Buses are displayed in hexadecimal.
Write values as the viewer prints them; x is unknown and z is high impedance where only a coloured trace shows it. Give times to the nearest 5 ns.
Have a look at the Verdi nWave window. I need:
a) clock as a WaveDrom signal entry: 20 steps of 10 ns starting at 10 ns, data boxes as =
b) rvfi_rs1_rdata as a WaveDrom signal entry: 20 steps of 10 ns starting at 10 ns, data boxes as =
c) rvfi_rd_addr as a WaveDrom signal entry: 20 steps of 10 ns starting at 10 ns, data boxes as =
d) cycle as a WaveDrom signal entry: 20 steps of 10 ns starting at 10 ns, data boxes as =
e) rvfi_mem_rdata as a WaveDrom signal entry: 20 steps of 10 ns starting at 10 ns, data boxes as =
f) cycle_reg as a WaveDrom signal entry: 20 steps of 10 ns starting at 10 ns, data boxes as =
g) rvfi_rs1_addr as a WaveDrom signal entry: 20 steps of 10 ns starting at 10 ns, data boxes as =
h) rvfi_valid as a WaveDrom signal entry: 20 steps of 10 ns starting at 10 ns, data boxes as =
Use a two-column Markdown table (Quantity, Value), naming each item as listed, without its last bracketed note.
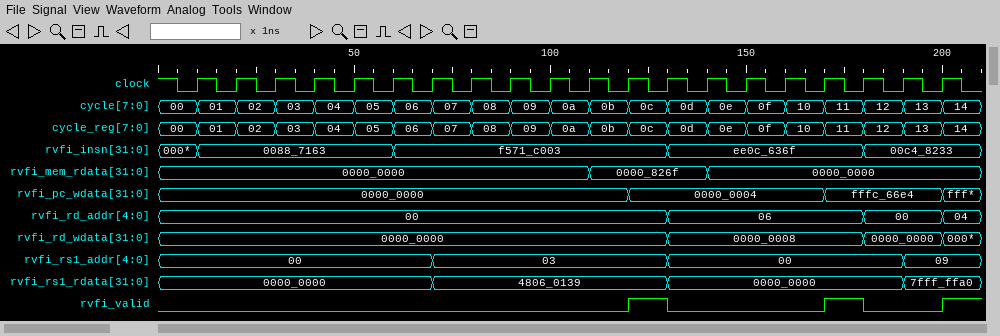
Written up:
| Quantity | Value |
|---|---|
| clock as a WaveDrom signal entry: 20 steps of 10 ns starting at 10 ns, data boxes as = | {name: 'clock', wave: 'p...................'} |
| rvfi_rs1_rdata as a WaveDrom signal entry: 20 steps of 10 ns starting at 10 ns, data boxes as = | {name: 'rvfi_rs1_rdata', wave: '=.....=.....=.....=.', data: '0000_0000 4806_0139 0000_0000 7fff_ffa0'} |
| rvfi_rd_addr as a WaveDrom signal entry: 20 steps of 10 ns starting at 10 ns, data boxes as = | {name: 'rvfi_rd_addr', wave: '=...........=....=.=', data: '00 06 00 04'} |
| cycle as a WaveDrom signal entry: 20 steps of 10 ns starting at 10 ns, data boxes as = | {name: 'cycle', wave: '====================', data: '01 02 03 04 05 06 07 08 09 0a 0b 0c 0d 0e 0f 10 11 12 13 14'} |
| rvfi_mem_rdata as a WaveDrom signal entry: 20 steps of 10 ns starting at 10 ns, data boxes as = | {name: 'rvfi_mem_rdata', wave: '=.........=..=......', data: '0000_0000 0000_826f 0000_0000'} |
| cycle_reg as a WaveDrom signal entry: 20 steps of 10 ns starting at 10 ns, data boxes as = | {name: 'cycle_reg', wave: '====================', data: '01 02 03 04 05 06 07 08 09 0a 0b 0c 0d 0e 0f 10 11 12 13 14'} |
| rvfi_rs1_addr as a WaveDrom signal entry: 20 steps of 10 ns starting at 10 ns, data boxes as = | {name: 'rvfi_rs1_addr', wave: '=.....=.....=.....=.', data: '00 03 00 09'} |
| rvfi_valid as a WaveDrom signal entry: 20 steps of 10 ns starting at 10 ns, data boxes as = | {name: 'rvfi_valid', wave: '0..........10...10.1'} |
